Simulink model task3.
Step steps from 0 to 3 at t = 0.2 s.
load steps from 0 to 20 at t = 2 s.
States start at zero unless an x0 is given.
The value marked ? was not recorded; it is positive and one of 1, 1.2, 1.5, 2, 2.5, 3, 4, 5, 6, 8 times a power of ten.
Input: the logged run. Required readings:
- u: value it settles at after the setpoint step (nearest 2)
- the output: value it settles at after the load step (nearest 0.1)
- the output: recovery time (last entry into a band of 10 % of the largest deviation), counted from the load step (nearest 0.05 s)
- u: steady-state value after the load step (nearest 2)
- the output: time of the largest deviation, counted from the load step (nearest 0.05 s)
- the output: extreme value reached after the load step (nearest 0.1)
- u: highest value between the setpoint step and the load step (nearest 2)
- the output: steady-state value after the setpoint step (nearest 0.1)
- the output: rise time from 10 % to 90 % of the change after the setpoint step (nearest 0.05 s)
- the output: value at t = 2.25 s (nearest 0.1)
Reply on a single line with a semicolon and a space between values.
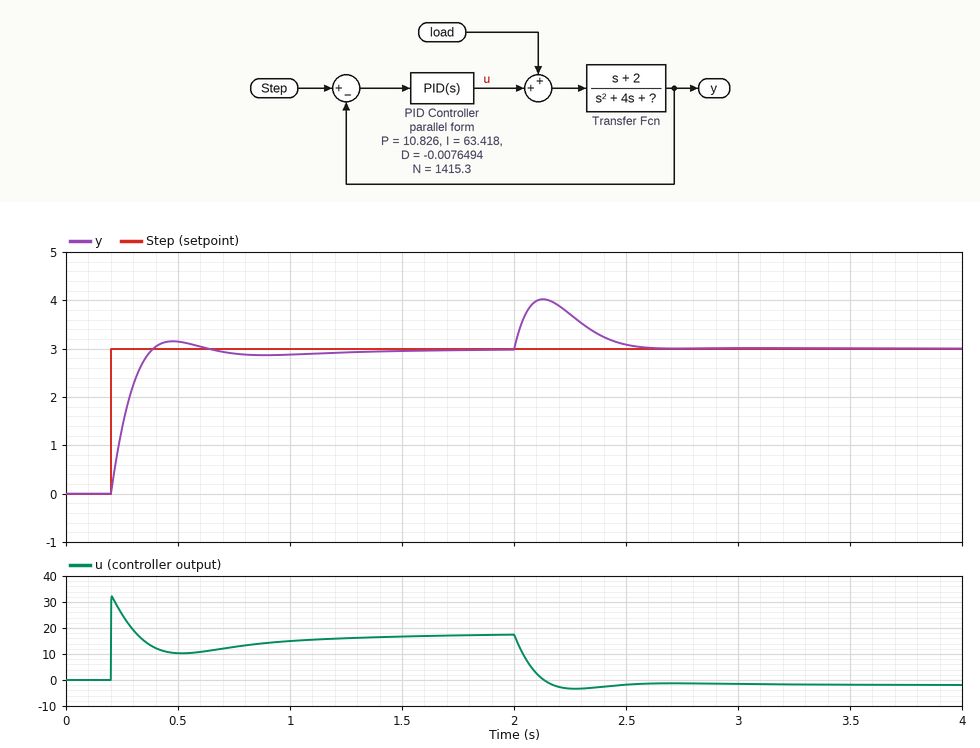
18; 3.0; 0.50 s; -2; 0.15 s; 4.0; 32; 3.0; 0.15 s; 3.7
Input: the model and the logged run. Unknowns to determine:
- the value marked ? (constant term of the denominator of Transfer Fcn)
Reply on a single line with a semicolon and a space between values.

12
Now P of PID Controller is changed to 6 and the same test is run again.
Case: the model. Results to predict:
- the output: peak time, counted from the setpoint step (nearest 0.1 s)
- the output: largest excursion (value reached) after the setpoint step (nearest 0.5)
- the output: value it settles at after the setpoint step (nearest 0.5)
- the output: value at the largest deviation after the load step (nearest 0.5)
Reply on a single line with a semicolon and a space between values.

0.3 s; 3.5; 3.0; 4.5
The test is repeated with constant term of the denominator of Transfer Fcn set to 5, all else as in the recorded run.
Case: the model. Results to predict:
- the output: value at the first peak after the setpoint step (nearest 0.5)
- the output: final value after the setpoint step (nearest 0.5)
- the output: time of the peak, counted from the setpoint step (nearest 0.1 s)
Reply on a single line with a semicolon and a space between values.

3.5; 3.0; 0.3 s
